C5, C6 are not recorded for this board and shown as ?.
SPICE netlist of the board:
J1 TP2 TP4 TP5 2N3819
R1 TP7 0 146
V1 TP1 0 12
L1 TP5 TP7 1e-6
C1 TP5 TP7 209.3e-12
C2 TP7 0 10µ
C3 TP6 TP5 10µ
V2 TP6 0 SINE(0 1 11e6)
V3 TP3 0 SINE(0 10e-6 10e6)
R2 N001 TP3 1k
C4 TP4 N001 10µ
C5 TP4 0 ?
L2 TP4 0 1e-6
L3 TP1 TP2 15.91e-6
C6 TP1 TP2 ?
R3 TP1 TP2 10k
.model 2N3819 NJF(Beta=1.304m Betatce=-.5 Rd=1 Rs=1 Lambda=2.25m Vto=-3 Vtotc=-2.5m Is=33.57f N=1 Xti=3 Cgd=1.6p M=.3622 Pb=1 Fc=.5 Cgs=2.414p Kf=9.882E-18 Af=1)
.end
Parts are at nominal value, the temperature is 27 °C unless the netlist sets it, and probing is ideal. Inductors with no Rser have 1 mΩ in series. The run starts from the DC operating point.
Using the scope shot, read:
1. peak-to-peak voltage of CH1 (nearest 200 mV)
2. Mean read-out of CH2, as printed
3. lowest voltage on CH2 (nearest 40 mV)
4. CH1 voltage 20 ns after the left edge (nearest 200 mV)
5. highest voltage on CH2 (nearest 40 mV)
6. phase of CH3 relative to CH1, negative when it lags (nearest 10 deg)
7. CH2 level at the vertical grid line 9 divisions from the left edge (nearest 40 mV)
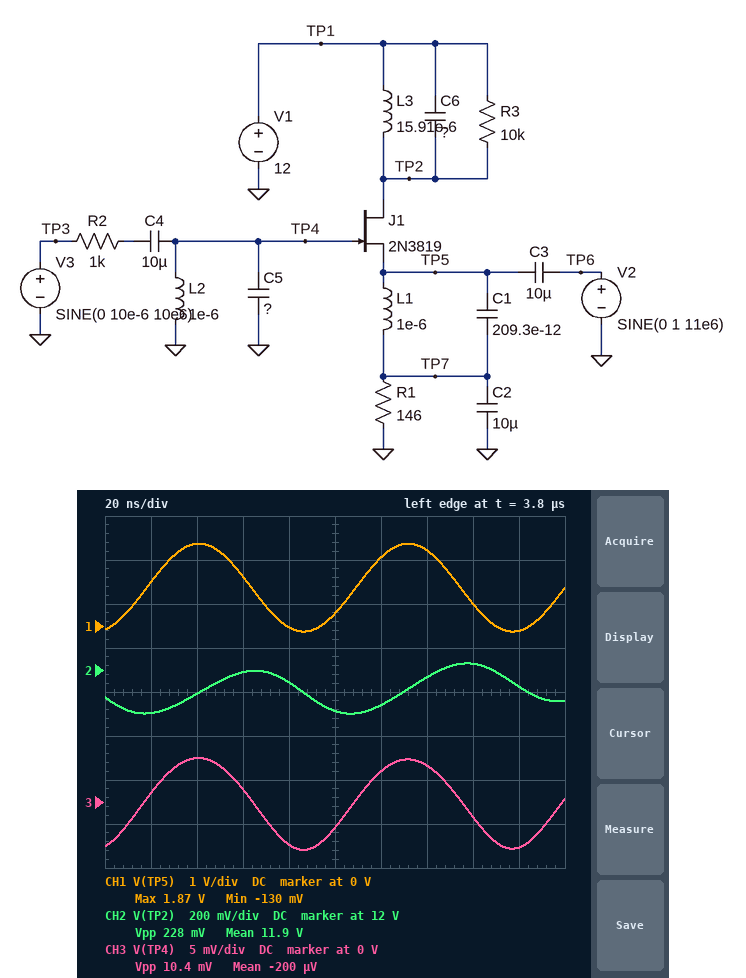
2.0 V
11.9 V
11.80 V
1.0 V
12.04 V
0 deg
11.92 V
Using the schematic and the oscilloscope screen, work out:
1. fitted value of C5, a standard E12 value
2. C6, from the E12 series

560 pF
820 pF
